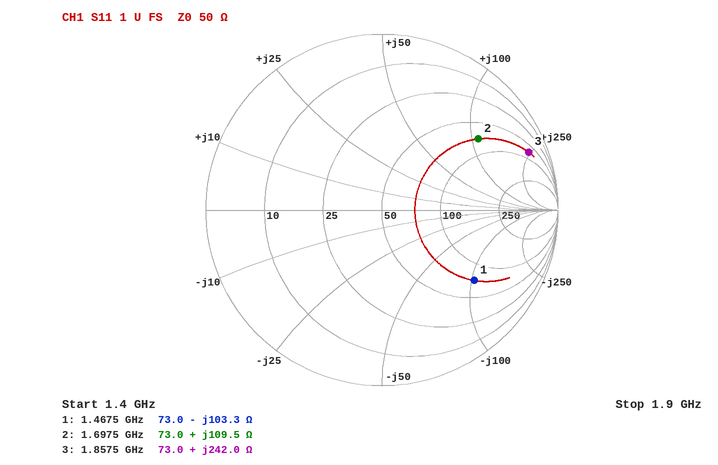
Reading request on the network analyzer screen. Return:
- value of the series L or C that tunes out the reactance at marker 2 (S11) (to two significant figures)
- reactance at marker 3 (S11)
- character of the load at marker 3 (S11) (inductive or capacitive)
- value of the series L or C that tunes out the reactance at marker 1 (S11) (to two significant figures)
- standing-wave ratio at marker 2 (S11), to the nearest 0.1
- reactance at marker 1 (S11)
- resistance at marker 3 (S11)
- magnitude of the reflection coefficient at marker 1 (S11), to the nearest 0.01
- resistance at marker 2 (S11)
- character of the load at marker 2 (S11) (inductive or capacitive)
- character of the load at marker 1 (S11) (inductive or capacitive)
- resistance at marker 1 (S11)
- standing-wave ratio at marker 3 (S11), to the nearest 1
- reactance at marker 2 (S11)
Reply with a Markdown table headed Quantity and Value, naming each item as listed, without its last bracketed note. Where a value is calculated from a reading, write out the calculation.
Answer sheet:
| Quantity | Value |
|---|---|
| value of the series L or C that tunes out the reactance at marker 2 (S11) | C = 1/(2π × 1.6975 GHz × 109.5 Ω) ≈ 856 fF, so 860 fF to two significant figures |
| reactance at marker 3 | +242.0 Ω |
| character of the load at marker 3 (S11) | inductive |
| value of the series L or C that tunes out the reactance at marker 1 (S11) | L = 103.3 Ω/(2π × 1.4675 GHz) ≈ 11 nH |
| standing-wave ratio at marker 2 (S11), to the nearest 0.1 | 5.2 |
| reactance at marker 1 | -103.3 Ω |
| resistance at marker 3 | 73.0 Ω |
| magnitude of the reflection coefficient at marker 1 (S11), to the nearest 0.01 | 0.66 |
| resistance at marker 2 | 73.0 Ω |
| character of the load at marker 2 (S11) | inductive |
| character of the load at marker 1 (S11) | capacitive |
| resistance at marker 1 | 73.0 Ω |
| standing-wave ratio at marker 3 (S11), to the nearest 1 | 18 |
| reactance at marker 2 | +109.5 Ω |
